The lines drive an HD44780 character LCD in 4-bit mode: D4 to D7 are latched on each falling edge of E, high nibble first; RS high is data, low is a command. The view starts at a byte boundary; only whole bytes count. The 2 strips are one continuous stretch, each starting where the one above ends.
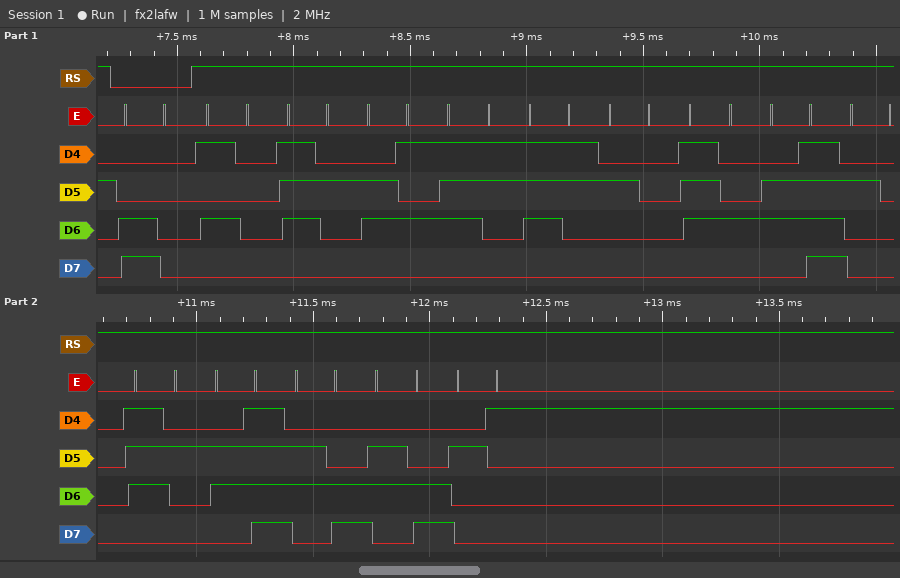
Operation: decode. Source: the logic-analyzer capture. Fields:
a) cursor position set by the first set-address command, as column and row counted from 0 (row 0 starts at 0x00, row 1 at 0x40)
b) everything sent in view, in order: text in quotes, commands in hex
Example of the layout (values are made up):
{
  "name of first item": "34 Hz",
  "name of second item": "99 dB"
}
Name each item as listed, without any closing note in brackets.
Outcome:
{
  "cursor position set by the first set-address command, as column and row counted from 0": "column 0, row 1",
  "everything sent in view, in order: text in quotes, commands in hex": "0xC0 \"Press to roll!\""
}
